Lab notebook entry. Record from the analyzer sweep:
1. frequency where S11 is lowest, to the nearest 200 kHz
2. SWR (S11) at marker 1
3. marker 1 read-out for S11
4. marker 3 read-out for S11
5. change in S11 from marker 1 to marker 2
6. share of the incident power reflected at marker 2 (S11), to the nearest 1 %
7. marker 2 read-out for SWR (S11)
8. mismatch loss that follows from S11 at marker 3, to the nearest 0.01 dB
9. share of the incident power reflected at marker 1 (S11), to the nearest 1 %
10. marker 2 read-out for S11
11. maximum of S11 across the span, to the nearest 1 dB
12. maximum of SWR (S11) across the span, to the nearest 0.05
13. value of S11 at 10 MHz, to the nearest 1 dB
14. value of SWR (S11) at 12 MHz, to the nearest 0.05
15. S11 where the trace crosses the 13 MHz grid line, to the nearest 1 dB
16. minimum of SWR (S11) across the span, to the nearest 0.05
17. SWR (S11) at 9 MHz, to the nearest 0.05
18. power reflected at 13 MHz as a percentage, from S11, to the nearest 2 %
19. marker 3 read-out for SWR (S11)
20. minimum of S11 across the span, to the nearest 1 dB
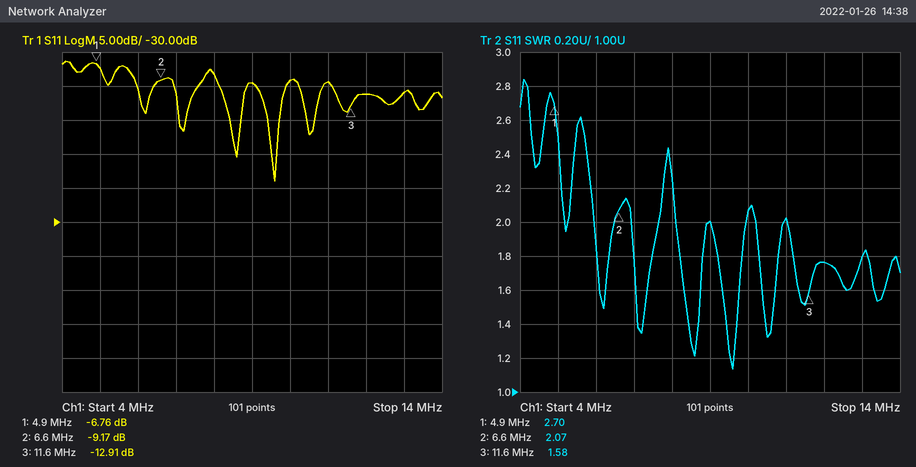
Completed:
9.6 MHz
2.70
-6.76 dB
-12.91 dB
-2.41 dB
12 %
2.07
0.23 dB
21 %
-9.17 dB
-6 dB
2.85
-9 dB
1.75
-11 dB
1.15
2.00
8 %
1.58
-24 dB
